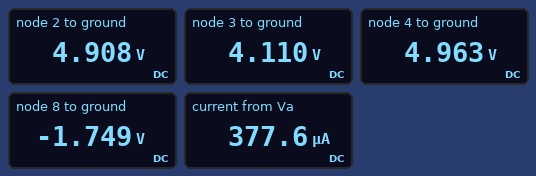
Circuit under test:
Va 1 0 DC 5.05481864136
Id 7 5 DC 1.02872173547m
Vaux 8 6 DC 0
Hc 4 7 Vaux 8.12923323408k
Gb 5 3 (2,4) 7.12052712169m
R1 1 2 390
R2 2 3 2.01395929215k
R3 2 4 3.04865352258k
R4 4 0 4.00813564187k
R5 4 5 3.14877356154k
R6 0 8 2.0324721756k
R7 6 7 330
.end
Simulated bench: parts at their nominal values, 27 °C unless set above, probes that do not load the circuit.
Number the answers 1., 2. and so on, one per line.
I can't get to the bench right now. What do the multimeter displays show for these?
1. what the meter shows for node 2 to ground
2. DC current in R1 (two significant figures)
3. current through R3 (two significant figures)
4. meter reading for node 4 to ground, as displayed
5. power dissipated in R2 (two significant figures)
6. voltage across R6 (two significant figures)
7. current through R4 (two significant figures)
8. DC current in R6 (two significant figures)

1. 4.908 V
2. 380 µA
3. 18 µA
4. 4.963 V
5. 320 µW
6. 1.7 V
7. 1.2 mA
8. 860 µA
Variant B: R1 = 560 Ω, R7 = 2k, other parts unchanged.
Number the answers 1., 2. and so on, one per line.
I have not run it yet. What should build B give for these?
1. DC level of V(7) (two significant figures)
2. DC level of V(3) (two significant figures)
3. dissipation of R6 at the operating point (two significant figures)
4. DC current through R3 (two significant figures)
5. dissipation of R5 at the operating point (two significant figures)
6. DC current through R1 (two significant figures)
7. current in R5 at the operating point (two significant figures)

1. -5.0 V
2. 5.0 V
3. 3.1 mW
4. 1.3 µA
5. 3.5 mW
6. 27 µA
7. 1.1 mA
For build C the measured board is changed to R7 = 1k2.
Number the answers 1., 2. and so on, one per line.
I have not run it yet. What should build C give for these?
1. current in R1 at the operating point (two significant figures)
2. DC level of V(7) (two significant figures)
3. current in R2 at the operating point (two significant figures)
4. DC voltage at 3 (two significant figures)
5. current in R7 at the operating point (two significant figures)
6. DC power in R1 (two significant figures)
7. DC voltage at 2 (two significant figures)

1. 230 µA
2. -3.3 V
3. 240 µA
4. 4.5 V
5. 1.0 mA
6. 20 µW
7. 5.0 V
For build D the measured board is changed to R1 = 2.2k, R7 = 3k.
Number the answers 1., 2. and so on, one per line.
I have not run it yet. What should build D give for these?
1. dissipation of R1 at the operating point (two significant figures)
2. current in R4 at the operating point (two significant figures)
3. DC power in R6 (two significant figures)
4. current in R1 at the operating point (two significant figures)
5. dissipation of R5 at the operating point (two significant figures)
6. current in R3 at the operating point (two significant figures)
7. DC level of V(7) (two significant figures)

1. 420 µW
2. 1.5 mA
3. 7.5 mW
4. 440 µA
5. 1.0 mW
6. 21 µA
7. -9.7 V
